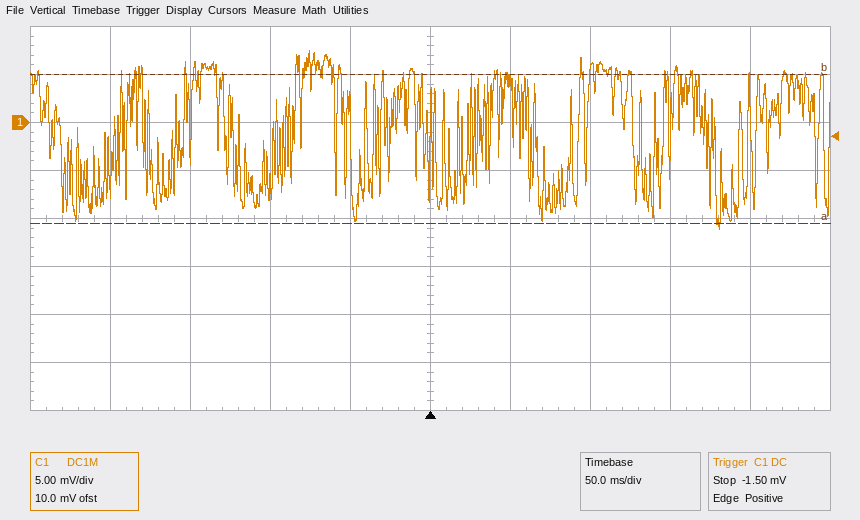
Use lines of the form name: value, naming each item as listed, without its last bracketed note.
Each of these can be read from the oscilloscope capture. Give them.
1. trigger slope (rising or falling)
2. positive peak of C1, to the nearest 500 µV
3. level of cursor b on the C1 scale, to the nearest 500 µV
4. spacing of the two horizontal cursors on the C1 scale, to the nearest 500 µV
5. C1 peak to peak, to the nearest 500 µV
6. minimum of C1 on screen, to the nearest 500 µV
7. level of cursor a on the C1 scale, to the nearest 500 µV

trigger slope: rising
positive peak of C1, to the nearest 500 µV: 7.5 mV
level of cursor b on the C1 scale, to the nearest 500 µV: 5.0 mV
spacing of the two horizontal cursors on the C1 scale, to the nearest 500 µV: 15.5 mV
C1 peak to peak, to the nearest 500 µV: 18.5 mV
minimum of C1 on screen, to the nearest 500 µV: -11.0 mV
level of cursor a on the C1 scale, to the nearest 500 µV: -10.5 mV
